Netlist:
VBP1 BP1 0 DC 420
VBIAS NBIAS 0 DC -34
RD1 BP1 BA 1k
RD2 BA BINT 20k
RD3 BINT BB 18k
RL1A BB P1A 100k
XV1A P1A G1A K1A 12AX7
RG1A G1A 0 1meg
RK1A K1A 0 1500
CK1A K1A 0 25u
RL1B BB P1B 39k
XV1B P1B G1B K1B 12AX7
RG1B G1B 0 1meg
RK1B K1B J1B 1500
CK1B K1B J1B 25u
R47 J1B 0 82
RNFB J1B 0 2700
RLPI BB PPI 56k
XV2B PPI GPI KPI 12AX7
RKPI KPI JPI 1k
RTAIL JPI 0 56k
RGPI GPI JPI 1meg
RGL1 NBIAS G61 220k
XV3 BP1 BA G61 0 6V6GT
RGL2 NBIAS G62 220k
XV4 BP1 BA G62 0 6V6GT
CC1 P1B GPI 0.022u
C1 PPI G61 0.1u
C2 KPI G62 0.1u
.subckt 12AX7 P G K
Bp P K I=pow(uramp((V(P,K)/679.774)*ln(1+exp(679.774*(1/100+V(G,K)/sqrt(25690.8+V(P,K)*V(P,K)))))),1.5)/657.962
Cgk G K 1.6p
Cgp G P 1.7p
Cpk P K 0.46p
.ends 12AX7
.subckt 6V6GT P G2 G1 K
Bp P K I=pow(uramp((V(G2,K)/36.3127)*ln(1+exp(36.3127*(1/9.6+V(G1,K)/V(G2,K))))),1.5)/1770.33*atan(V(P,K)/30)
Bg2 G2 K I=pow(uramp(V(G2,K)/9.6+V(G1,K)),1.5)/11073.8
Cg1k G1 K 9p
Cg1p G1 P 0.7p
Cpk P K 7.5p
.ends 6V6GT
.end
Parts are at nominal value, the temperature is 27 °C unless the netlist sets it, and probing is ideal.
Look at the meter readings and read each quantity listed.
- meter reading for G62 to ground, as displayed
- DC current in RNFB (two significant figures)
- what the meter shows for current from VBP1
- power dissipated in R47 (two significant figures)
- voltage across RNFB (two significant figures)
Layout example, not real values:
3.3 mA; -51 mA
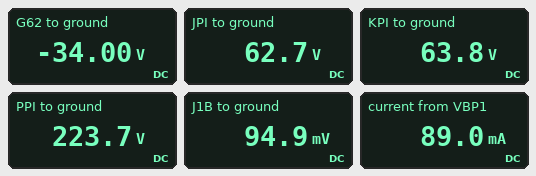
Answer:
-34.00 V; 35 µA; 89.0 mA; 110 µW; 95 mV
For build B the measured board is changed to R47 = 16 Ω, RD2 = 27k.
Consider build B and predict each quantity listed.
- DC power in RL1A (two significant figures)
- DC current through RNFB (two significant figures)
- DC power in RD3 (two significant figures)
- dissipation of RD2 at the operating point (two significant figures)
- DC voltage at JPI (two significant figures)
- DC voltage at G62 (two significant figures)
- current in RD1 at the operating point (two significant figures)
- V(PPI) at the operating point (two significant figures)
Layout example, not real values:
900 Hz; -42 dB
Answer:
88 mW; 6.8 µA; 180 mW; 270 mW; 59 V; -34 V; 8.0 mA; 210 V
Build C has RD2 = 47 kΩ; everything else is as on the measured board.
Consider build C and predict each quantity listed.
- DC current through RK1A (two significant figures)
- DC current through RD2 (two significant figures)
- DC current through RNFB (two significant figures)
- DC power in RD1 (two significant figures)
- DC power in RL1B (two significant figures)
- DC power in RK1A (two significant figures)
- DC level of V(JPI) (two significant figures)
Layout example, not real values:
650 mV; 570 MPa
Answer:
830 µA; 2.7 mA; 29 µA; 58 mW; 38 mW; 1.0 mW; 52 V
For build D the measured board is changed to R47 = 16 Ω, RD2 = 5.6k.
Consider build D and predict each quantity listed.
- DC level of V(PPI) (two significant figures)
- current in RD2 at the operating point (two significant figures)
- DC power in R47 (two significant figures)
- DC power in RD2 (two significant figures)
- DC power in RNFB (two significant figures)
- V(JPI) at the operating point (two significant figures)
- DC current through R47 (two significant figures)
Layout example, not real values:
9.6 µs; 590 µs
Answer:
250 V; 3.7 mA; 30 µW; 78 mW; 180 nW; 70 V; 1.4 mA
